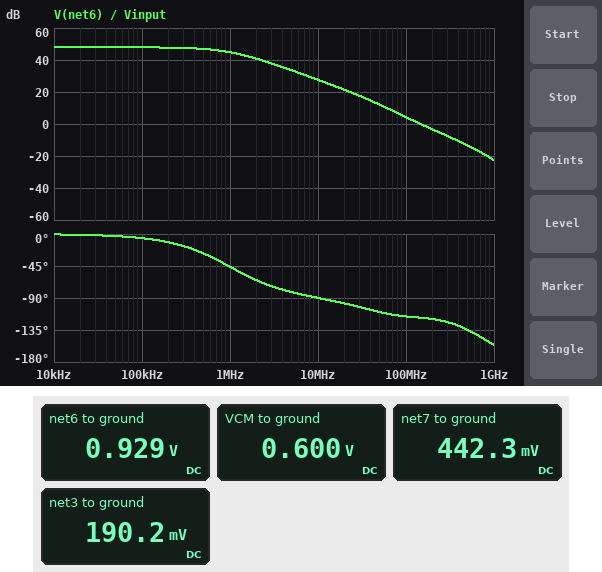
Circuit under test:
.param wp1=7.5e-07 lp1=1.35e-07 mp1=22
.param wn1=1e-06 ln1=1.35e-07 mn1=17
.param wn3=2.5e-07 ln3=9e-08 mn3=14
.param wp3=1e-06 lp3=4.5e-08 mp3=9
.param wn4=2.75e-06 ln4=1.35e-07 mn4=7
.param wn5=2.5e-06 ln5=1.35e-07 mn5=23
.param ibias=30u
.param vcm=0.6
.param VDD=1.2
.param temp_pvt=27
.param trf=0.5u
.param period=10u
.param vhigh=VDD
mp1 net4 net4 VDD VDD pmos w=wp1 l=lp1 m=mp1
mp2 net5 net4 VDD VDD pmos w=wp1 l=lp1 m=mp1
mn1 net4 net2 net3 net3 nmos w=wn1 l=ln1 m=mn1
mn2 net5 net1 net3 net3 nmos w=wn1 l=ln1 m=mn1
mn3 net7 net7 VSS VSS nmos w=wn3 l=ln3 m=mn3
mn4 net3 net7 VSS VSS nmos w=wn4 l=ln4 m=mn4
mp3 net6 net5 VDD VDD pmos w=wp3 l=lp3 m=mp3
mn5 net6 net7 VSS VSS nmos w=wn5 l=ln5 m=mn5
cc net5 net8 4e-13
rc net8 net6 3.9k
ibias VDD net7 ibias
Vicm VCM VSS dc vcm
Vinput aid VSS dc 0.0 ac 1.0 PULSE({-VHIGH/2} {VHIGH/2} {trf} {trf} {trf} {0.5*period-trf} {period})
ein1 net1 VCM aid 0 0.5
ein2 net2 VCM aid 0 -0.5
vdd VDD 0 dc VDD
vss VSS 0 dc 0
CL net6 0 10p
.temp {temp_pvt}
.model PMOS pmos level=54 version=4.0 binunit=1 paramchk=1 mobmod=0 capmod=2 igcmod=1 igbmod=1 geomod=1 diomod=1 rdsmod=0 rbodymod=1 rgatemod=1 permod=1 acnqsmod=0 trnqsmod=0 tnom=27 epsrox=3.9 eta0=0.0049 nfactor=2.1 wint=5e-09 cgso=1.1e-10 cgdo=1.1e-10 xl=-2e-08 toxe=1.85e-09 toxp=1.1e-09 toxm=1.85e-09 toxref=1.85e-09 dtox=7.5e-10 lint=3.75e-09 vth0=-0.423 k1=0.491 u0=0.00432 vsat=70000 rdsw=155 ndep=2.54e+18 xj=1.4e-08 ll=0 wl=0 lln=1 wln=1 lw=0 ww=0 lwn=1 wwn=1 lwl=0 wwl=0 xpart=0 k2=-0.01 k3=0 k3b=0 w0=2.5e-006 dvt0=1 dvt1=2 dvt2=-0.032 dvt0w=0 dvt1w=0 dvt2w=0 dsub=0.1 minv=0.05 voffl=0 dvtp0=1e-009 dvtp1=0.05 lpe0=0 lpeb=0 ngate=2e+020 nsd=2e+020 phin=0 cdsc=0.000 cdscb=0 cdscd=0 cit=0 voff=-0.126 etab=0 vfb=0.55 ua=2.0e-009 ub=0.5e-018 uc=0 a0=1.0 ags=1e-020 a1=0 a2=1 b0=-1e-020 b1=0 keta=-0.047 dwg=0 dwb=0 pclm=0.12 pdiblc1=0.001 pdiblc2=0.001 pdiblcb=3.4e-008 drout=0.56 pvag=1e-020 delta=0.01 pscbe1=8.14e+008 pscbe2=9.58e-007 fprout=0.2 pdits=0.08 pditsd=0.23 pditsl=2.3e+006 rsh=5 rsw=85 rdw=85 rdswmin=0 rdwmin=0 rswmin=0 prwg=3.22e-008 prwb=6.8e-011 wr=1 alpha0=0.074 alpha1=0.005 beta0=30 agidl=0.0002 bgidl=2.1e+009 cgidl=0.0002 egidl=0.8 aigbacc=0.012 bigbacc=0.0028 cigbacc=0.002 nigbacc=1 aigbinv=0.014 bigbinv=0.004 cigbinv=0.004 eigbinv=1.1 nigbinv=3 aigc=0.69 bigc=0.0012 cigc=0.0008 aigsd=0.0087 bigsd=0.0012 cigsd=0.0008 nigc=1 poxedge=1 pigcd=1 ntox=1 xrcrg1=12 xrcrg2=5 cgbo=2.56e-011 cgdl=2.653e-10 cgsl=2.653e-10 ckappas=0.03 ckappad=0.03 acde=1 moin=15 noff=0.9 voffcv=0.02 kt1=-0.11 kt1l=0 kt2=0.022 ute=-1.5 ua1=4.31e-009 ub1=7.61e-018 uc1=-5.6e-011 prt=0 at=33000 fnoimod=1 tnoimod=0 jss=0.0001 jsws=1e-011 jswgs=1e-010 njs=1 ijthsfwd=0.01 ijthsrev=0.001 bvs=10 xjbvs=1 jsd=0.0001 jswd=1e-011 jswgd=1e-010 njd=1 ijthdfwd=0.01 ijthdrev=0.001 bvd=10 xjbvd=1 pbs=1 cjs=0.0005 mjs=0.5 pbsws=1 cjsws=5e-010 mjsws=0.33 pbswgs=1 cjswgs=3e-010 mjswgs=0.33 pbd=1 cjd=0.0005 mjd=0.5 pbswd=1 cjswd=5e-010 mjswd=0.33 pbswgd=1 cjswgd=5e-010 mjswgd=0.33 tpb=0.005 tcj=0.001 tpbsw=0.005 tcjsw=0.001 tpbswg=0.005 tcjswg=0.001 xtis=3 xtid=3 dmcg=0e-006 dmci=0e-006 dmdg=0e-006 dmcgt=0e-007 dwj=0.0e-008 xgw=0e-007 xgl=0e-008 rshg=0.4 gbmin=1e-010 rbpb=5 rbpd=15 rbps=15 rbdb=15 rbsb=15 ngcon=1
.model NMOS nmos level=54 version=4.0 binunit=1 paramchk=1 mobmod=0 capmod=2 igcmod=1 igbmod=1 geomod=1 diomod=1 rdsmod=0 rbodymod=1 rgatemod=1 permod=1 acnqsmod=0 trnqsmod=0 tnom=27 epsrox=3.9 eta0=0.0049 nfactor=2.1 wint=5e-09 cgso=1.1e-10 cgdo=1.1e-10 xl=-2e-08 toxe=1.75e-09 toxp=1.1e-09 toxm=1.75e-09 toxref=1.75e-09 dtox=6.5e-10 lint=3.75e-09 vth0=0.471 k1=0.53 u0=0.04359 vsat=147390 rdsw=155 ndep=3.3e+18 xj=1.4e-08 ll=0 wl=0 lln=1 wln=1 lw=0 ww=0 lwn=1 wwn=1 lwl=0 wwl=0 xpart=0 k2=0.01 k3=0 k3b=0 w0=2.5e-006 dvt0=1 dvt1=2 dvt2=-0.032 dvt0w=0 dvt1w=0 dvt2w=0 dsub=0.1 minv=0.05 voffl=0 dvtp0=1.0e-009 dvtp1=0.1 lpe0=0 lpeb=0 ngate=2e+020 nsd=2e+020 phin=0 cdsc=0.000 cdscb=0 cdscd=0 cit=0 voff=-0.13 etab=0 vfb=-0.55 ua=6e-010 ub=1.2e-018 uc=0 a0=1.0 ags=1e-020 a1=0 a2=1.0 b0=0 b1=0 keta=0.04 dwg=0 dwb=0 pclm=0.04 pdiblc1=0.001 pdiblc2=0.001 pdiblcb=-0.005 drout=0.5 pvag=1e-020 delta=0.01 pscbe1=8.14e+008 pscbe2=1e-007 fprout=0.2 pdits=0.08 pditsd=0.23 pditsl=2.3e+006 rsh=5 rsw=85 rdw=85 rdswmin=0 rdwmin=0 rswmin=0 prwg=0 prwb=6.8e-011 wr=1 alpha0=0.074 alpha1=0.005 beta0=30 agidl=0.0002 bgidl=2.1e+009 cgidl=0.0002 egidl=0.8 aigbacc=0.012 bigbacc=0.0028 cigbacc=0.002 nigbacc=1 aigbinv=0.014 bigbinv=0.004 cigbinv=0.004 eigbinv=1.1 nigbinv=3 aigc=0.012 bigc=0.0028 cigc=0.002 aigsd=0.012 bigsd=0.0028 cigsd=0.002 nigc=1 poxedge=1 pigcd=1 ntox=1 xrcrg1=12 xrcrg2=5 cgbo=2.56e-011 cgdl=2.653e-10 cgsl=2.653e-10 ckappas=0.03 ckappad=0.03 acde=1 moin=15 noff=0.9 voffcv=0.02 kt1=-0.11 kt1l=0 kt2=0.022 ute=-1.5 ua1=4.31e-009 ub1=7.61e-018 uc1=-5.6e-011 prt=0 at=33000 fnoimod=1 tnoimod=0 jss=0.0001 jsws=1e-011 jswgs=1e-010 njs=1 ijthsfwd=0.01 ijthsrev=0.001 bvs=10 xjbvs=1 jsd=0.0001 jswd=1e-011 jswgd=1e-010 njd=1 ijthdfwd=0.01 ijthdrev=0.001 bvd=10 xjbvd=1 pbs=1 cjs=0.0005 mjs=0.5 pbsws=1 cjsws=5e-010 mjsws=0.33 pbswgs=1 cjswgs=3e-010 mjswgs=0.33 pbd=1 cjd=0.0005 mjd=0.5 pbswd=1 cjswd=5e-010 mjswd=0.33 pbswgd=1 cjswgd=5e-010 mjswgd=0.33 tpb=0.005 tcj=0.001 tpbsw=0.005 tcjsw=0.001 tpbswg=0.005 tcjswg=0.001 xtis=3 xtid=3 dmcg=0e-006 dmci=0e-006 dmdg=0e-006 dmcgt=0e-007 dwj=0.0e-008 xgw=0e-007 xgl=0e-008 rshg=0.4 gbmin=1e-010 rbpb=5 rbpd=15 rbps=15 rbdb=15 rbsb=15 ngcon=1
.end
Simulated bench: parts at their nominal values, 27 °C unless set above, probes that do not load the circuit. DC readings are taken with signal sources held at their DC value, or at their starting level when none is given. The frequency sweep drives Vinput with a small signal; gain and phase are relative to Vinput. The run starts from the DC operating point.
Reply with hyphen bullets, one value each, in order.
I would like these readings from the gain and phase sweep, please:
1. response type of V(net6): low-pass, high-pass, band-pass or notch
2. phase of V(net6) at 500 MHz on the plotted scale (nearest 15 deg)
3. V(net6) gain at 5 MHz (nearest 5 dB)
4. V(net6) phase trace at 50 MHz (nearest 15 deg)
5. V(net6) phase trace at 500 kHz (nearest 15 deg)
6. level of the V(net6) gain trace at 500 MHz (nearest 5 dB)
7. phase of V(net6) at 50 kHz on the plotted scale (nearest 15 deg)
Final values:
- low-pass
- -135 deg
- 35 dB
- -105 deg
- -30 deg
- -15 dB
- 0 deg
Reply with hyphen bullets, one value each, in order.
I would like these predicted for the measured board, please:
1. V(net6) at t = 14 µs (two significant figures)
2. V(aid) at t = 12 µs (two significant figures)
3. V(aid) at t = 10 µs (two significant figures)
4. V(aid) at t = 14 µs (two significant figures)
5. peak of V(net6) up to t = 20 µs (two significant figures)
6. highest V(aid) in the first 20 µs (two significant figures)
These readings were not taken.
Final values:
- 1.2 V
- 600 mV
- -600 mV
- 600 mV
- 1.2 V
- 600 mV
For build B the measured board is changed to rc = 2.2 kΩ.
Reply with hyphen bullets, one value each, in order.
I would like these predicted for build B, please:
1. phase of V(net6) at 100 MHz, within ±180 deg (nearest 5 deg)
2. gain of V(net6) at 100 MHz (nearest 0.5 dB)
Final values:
- -130 deg
- 2.5 dB
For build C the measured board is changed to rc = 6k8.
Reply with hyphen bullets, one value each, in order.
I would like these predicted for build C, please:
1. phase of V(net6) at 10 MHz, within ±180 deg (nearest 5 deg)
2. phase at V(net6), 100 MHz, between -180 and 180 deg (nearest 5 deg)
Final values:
- -85 deg
- -105 deg
